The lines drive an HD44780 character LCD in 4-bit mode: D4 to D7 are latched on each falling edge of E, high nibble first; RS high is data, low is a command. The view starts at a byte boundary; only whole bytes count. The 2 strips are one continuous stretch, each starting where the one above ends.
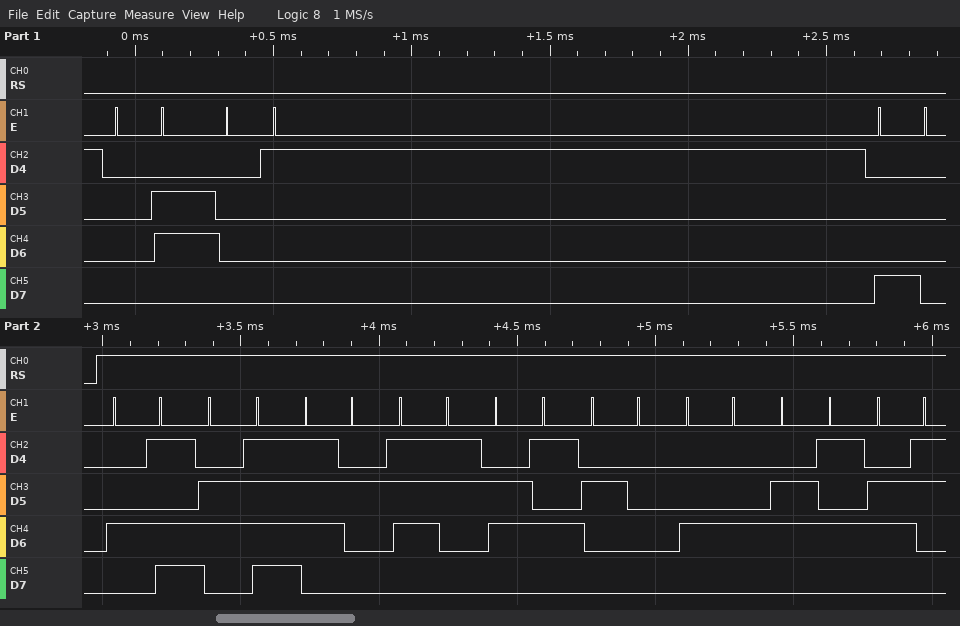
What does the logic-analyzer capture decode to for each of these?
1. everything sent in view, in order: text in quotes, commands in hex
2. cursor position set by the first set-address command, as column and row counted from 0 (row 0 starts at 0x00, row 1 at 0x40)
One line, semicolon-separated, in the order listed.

0x06 0x01 0x80 "Morse Dec"; column 0, row 0
